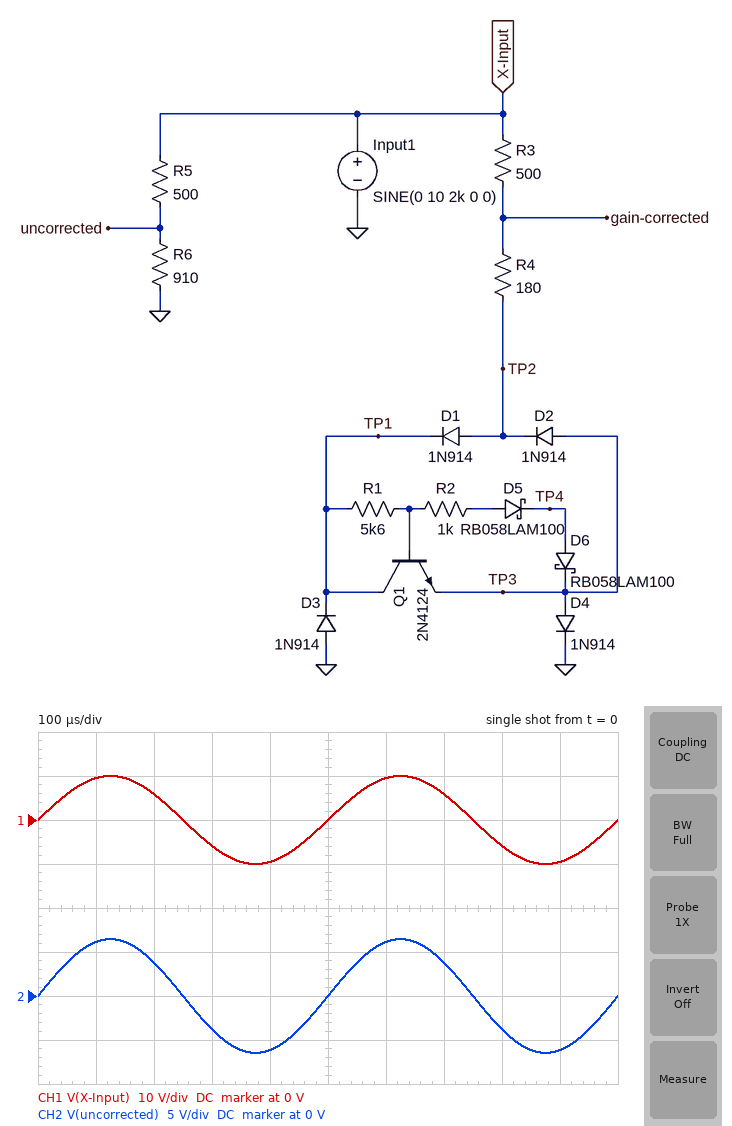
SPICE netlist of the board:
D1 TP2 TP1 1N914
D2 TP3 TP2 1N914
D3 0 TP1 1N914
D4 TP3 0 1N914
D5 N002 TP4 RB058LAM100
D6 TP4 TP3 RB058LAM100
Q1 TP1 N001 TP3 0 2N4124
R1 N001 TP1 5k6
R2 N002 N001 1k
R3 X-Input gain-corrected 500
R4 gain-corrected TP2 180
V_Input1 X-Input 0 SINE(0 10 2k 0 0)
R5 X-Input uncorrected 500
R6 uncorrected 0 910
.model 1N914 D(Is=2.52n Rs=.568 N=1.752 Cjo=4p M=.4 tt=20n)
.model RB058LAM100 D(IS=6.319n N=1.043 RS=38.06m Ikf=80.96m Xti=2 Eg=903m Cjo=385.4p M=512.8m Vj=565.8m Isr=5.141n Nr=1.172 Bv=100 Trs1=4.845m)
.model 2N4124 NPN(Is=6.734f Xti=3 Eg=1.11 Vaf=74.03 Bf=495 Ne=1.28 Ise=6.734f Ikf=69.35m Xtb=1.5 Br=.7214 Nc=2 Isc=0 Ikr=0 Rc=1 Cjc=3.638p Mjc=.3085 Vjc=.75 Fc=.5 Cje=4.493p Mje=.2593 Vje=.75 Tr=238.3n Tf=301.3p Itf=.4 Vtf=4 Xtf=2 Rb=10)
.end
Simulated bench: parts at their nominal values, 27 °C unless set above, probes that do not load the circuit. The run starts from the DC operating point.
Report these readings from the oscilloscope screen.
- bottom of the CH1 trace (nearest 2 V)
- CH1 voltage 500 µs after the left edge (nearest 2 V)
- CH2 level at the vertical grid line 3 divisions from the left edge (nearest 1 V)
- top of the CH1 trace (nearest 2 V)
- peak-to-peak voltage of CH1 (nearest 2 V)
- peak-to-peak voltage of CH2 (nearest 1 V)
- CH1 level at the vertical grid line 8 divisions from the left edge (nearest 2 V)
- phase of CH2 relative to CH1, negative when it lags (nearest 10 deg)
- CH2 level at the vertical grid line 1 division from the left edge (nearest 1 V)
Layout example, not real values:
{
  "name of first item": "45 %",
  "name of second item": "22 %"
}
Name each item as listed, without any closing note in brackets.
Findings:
{
  "bottom of the CH1 trace": "-10 V",
  "CH1 voltage 500 µs after the left edge": "0 V",
  "CH2 level at the vertical grid line 3 divisions from the left edge": "-4 V",
  "top of the CH1 trace": "10 V",
  "peak-to-peak voltage of CH1": "20 V",
  "peak-to-peak voltage of CH2": "13 V",
  "CH1 level at the vertical grid line 8 divisions from the left edge": "-6 V",
  "phase of CH2 relative to CH1, negative when it lags": "0 deg",
  "CH2 level at the vertical grid line 1 division from the left edge": "6 V"
}
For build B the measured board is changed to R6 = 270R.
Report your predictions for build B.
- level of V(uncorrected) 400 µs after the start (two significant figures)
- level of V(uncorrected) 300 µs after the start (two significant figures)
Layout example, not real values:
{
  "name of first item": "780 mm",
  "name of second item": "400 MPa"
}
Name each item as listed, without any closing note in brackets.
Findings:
{
  "level of V(uncorrected) 400 µs after the start": "-3.3 V",
  "level of V(uncorrected) 300 µs after the start": "-2.1 V"
}
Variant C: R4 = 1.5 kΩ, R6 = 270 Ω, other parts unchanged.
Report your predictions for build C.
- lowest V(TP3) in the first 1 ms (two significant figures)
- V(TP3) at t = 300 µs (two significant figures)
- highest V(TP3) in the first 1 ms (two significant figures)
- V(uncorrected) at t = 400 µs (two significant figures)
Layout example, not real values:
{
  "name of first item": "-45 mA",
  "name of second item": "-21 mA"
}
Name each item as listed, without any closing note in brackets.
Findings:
{
  "lowest V(TP3) in the first 1 ms": "-2.3 V",
  "V(TP3) at t = 300 µs": "-2.1 V",
  "highest V(TP3) in the first 1 ms": "640 mV",
  "V(uncorrected) at t = 400 µs": "-3.3 V"
}
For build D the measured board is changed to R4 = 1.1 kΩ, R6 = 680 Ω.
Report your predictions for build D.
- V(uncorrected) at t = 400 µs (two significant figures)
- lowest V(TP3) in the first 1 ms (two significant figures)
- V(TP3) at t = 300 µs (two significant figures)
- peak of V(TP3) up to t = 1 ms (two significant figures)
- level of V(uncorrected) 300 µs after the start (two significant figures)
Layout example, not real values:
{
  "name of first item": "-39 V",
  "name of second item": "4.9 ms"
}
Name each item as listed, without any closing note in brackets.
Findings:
{
  "V(uncorrected) at t = 400 µs": "-5.5 V",
  "lowest V(TP3) in the first 1 ms": "-2.4 V",
  "V(TP3) at t = 300 µs": "-2.2 V",
  "peak of V(TP3) up to t = 1 ms": "650 mV",
  "level of V(uncorrected) 300 µs after the start": "-3.4 V"
}
